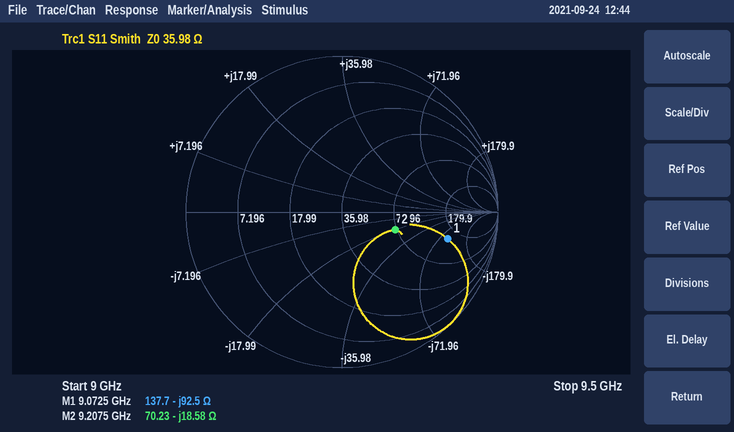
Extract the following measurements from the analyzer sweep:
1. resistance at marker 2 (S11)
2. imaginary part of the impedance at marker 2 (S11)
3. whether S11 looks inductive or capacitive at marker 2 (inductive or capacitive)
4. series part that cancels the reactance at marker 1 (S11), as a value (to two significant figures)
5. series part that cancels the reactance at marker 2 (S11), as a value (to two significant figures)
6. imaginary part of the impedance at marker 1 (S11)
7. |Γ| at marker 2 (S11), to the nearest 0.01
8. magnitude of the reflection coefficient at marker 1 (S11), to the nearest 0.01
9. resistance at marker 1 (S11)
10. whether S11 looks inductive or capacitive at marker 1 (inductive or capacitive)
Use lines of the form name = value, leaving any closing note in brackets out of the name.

resistance at marker 2 = 70.23 Ω
imaginary part of the impedance at marker 2 = -18.58 Ω
whether S11 looks inductive or capacitive at marker 2 = capacitive
series part that cancels the reactance at marker 1 (S11), as a value = 1.6 nH
series part that cancels the reactance at marker 2 (S11), as a value = 320 pH
imaginary part of the impedance at marker 1 = -92.5 Ω
|Γ| at marker 2 (S11), to the nearest 0.01 = 0.36
magnitude of the reflection coefficient at marker 1 (S11), to the nearest 0.01 = 0.70
resistance at marker 1 = 137.7 Ω
whether S11 looks inductive or capacitive at marker 1 = capacitive
